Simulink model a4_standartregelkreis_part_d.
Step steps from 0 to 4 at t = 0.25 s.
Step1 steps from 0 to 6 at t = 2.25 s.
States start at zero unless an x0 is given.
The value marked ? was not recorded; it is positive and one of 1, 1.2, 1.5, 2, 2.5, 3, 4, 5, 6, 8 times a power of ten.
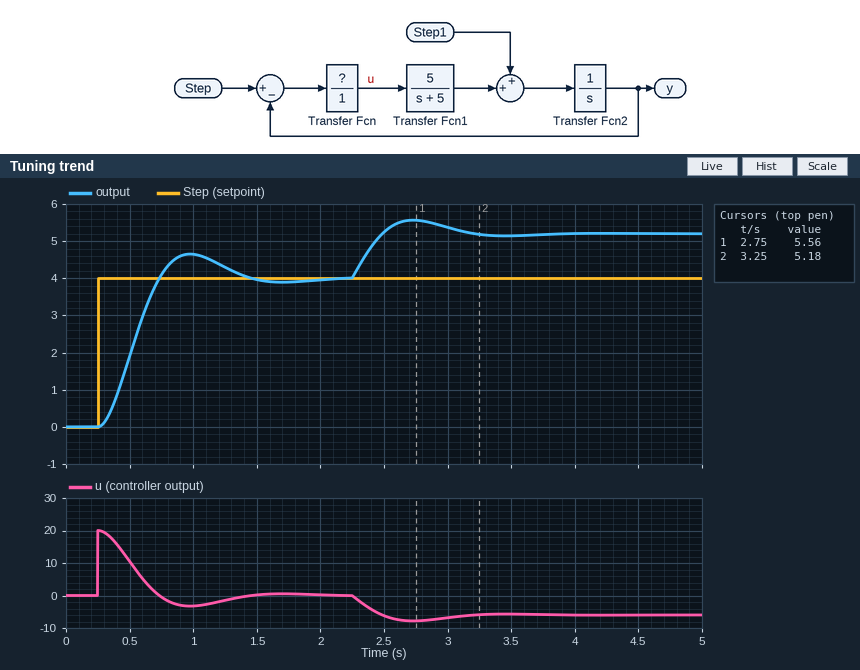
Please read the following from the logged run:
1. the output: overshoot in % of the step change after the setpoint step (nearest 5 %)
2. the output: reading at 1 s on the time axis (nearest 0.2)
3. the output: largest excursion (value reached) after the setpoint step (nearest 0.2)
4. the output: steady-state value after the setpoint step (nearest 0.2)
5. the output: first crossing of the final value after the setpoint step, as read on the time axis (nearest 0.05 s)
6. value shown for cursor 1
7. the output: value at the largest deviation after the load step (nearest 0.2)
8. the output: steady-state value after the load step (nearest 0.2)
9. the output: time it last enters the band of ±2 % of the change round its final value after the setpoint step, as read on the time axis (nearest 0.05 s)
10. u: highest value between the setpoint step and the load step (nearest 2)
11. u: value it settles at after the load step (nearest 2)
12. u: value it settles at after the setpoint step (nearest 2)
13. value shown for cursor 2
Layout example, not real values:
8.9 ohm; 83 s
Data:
15 %; 4.6; 4.6; 4.0; 0.75 s; 5.56; 5.6; 5.2; 1.85 s; 20; -6; 0; 5.18
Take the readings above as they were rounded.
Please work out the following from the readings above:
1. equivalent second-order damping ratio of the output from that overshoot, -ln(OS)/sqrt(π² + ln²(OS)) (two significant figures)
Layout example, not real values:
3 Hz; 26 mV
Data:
0.52
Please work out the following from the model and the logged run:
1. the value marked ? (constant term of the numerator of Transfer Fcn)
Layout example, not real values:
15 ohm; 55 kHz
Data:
5
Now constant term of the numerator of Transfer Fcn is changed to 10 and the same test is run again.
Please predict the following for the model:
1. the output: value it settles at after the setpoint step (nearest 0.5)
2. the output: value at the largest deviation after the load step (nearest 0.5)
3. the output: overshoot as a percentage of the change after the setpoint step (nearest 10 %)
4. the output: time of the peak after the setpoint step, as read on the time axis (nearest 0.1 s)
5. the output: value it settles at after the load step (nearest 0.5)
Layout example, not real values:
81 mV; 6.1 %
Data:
4.0; 5.0; 30 %; 0.7 s; 4.5
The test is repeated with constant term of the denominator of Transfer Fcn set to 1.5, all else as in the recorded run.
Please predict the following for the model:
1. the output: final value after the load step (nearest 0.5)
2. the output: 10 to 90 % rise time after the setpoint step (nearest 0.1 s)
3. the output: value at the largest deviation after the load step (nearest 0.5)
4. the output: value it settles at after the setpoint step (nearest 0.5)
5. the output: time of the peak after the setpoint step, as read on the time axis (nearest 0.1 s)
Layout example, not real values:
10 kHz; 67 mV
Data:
6.0; 0.5 s; 6.0; 4.0; 1.2 s
